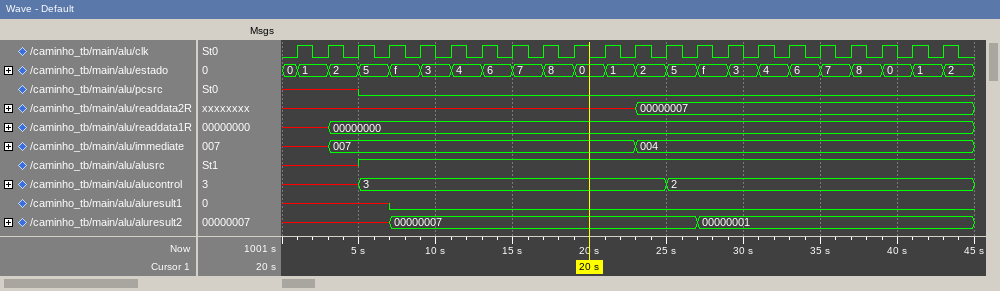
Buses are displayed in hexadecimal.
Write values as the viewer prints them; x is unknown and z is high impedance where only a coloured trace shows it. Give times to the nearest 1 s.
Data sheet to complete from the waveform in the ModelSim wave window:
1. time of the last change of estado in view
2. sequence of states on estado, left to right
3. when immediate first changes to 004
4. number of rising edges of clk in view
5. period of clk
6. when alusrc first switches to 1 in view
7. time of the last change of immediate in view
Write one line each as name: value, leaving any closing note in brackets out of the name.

time of the last change of estado in view: 43 s
sequence of states on estado, left to right: 0, 1, 2, 5, f, 3, 4, 6, 7, 8, 0, 1, 2, 5, f, 3, 4, 6, 7, 8, 0, 1, 2
when immediate first changes to 004: 23 s
number of rising edges of clk in view: 22
period of clk: 2 s
when alusrc first switches to 1 in view: 5 s
time of the last change of immediate in view: 23 s
